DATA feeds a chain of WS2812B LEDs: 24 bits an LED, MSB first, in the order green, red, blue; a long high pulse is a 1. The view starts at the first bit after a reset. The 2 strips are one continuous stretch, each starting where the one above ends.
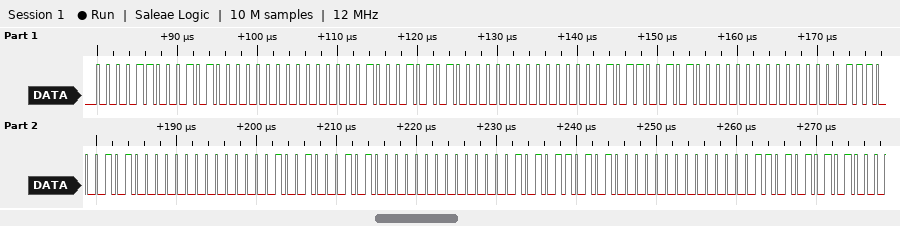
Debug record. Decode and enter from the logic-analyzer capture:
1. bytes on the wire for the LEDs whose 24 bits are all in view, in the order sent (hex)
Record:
0C 50 00 11 50 00 16 50 00 1C 50 00 24 50 00 2B 50 00
